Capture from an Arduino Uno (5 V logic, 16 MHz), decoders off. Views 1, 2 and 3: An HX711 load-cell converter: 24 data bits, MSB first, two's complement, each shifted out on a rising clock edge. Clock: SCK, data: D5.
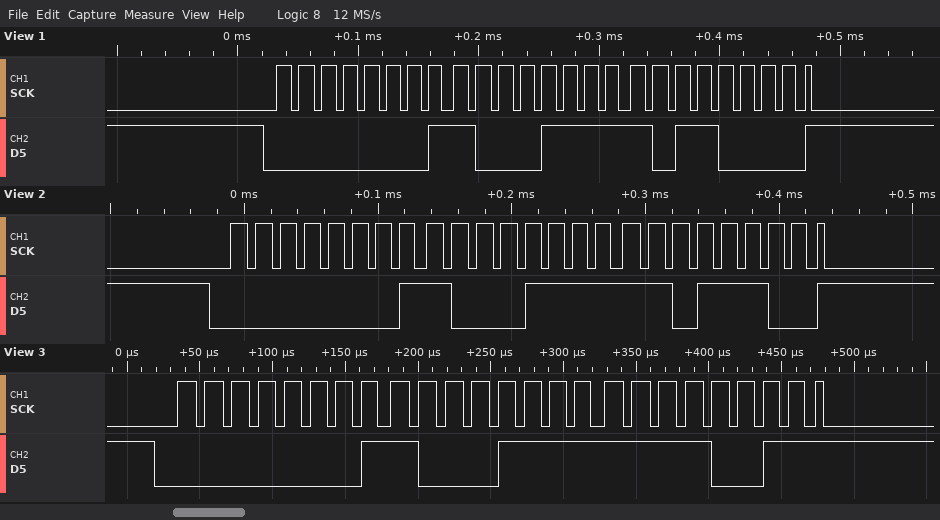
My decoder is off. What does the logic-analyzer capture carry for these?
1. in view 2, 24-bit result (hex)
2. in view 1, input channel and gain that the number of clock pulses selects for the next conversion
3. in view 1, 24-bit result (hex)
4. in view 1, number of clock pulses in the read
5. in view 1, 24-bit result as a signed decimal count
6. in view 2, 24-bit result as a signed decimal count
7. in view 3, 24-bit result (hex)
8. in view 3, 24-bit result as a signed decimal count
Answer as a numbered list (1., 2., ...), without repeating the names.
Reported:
1. 0x018FDC
2. channel A, gain 128
3. 0x018FB0
4. 25
5. 102320
6. 102364
7. 0x018FF3
8. 102387
